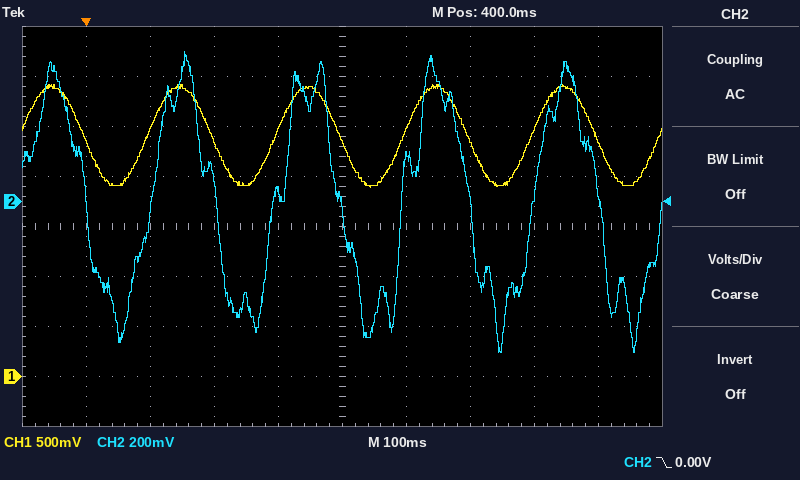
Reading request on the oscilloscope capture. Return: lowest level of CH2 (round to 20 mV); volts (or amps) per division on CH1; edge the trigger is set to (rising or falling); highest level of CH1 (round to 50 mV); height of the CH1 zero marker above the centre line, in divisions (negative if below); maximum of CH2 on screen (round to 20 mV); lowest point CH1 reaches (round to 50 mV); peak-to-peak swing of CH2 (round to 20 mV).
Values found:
-600 mV
500 mV
falling
2.90 V
-3.0 div
600 mV
1.90 V
1.20 V
